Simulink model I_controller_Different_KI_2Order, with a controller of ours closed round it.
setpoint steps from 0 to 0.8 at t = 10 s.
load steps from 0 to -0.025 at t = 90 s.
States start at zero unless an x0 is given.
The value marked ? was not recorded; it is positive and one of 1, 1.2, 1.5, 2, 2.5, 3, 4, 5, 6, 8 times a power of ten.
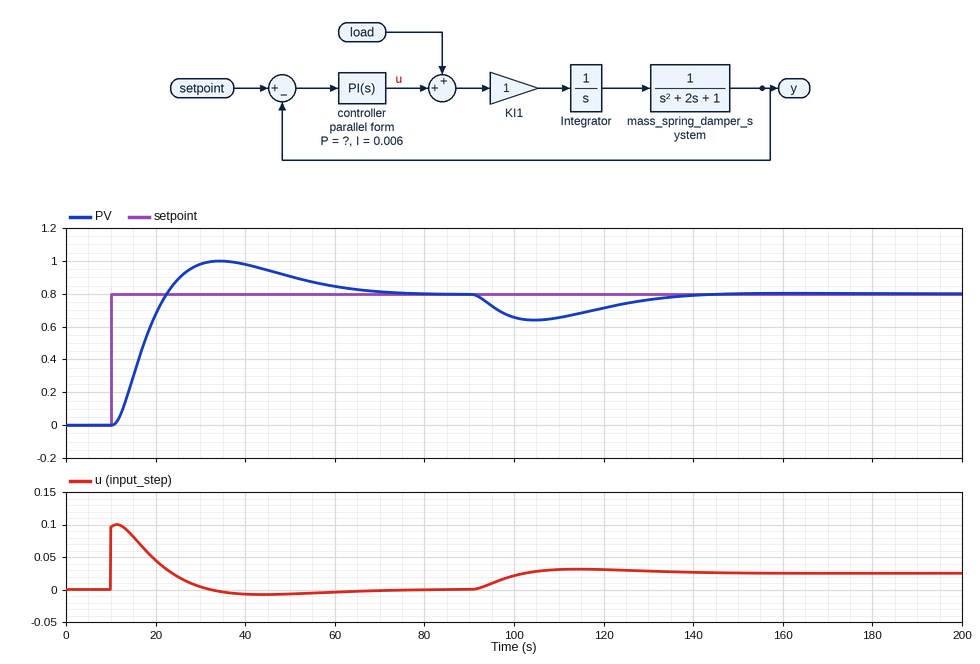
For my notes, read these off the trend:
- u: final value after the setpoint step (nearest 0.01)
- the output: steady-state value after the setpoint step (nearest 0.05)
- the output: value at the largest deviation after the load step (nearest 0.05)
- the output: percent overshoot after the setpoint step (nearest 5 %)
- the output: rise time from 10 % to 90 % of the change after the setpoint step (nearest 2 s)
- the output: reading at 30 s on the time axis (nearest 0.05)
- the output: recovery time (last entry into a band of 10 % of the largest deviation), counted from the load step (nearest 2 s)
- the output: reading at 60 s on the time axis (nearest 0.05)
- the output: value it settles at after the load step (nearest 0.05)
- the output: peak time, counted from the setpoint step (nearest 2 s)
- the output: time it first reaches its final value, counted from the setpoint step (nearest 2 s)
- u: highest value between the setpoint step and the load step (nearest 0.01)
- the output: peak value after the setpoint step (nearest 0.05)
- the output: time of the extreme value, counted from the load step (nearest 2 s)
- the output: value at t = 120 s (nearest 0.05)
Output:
0.00
0.80
0.65
25 %
8 s
1.00
48 s
0.85
0.80
24 s
12 s
0.10
1.00
14 s
0.70
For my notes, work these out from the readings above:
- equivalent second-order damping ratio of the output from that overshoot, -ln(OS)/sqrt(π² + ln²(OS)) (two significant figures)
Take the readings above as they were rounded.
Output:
0.40
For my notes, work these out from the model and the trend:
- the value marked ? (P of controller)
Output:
0.12
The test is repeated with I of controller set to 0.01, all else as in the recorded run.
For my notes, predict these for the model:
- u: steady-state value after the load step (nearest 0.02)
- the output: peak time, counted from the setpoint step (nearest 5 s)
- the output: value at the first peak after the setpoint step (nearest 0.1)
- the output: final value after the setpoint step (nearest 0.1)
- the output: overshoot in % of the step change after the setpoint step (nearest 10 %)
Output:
0.02
20 s
1.1
0.8
40 %
